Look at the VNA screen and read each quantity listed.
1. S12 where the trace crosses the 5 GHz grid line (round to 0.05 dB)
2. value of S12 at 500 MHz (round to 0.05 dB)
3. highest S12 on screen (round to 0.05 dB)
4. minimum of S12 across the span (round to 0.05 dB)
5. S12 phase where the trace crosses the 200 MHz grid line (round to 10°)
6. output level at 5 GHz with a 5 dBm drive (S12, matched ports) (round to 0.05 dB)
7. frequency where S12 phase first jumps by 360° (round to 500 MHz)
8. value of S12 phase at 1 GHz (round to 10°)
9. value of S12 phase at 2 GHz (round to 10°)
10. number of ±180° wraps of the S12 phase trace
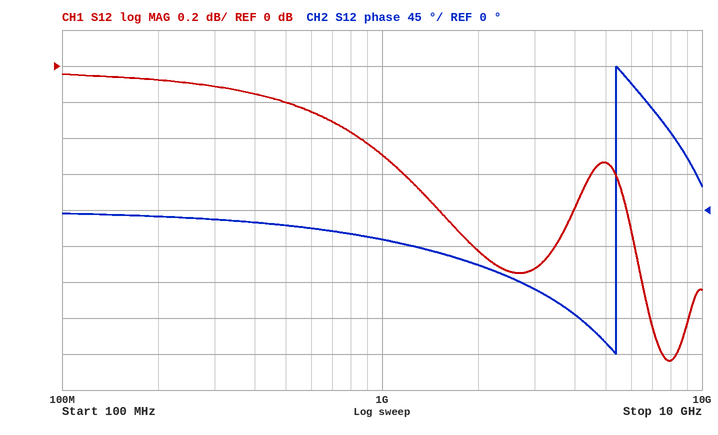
-0.55 dB
-0.20 dB
-0.05 dB
-1.65 dB
-10°
4.45 dBm
5.5 GHz
-40°
-70°
1
